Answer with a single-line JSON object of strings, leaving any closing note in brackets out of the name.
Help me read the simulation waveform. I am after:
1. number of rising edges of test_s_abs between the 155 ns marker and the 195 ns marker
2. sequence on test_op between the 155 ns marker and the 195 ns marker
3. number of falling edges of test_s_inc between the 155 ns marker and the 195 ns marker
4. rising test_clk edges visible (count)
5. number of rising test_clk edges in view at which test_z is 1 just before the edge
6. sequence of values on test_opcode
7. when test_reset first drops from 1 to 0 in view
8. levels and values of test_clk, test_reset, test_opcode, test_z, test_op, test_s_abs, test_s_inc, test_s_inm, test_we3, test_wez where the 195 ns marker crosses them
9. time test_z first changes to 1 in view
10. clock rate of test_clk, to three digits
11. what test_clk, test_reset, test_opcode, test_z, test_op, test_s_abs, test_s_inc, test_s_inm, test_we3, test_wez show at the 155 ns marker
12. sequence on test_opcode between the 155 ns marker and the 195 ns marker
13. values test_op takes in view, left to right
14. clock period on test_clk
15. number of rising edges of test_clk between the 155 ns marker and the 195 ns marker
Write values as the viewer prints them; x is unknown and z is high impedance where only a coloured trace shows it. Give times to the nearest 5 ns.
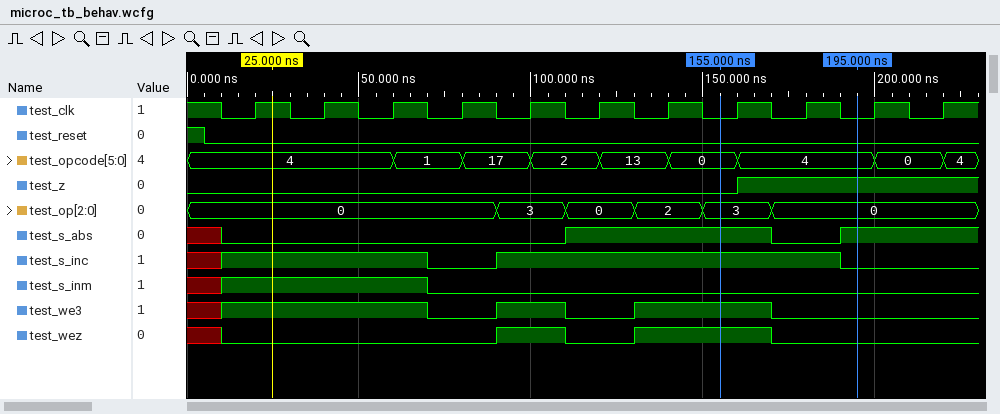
{"number of rising edges of test_s_abs between the 155 ns marker and the 195 ns marker": "1", "sequence on test_op between the 155 ns marker and the 195 ns marker": "3, 0", "number of falling edges of test_s_inc between the 155 ns marker and the 195 ns marker": "1", "rising test_clk edges visible": "11", "number of rising test_clk edges in view at which test_z is 1 just before the edge": "3", "sequence of values on test_opcode": "4, 1, 17, 2, 13, 0, 4, 0, 4", "when test_reset first drops from 1 to 0 in view": "5 ns", "levels and values of test_clk, test_reset, test_opcode, test_z, test_op, test_s_abs, test_s_inc, test_s_inm, test_we3, test_wez where the 195 ns marker crosses them": "test_clk=0, test_reset=0, test_opcode=4, test_z=1, test_op=0, test_s_abs=1, test_s_inc=0, test_s_inm=0, test_we3=0, test_wez=0", "time test_z first changes to 1 in view": "160 ns", "clock rate of test_clk, to three digits": "50.0 MHz", "what test_clk, test_reset, test_opcode, test_z, test_op, test_s_abs, test_s_inc, test_s_inm, test_we3, test_wez show at the 155 ns marker": "test_clk=0, test_reset=0, test_opcode=0, test_z=0, test_op=3, test_s_abs=1, test_s_inc=1, test_s_inm=0, test_we3=1, test_wez=1", "sequence on test_opcode between the 155 ns marker and the 195 ns marker": "0, 4", "values test_op takes in view, left to right": "0, 3, 0, 2, 3, 0", "clock period on test_clk": "20 ns", "number of rising edges of test_clk between the 155 ns marker and the 195 ns marker": "2"}
